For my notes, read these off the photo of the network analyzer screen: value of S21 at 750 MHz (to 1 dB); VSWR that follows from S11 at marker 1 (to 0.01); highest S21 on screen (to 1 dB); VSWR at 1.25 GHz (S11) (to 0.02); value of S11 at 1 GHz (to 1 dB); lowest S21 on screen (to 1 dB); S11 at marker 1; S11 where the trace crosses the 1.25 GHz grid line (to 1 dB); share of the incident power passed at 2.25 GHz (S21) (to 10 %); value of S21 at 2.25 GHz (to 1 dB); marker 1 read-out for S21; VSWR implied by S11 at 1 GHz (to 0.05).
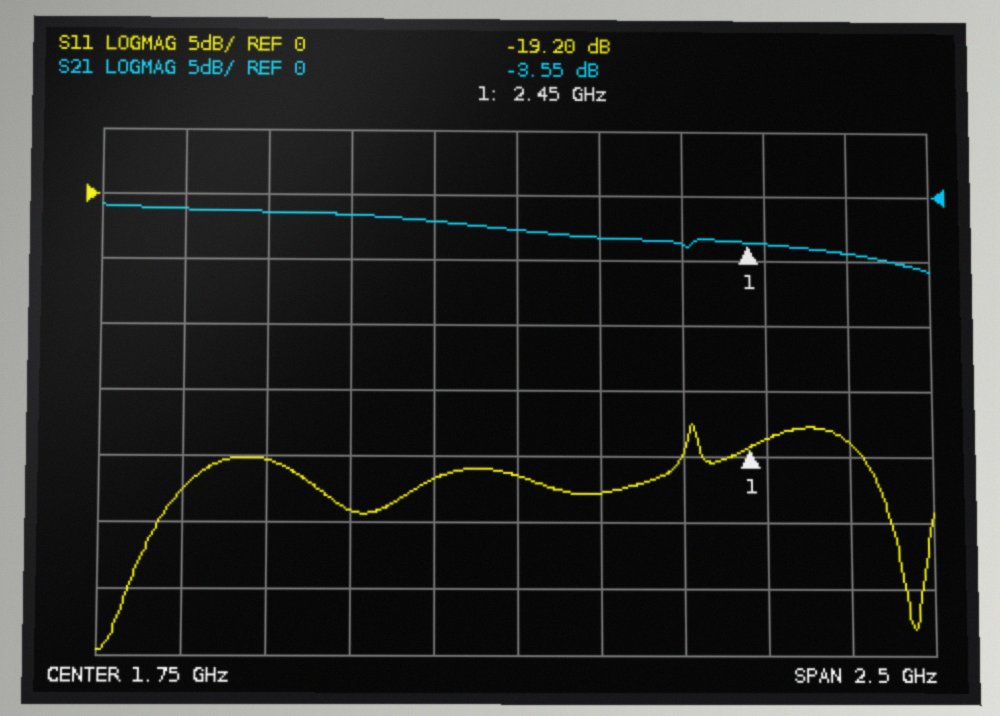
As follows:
-1 dB
1.25
-1 dB
1.14
-20 dB
-6 dB
-19.20 dB
-24 dB
40 %
-4 dB
-3.55 dB
1.20
